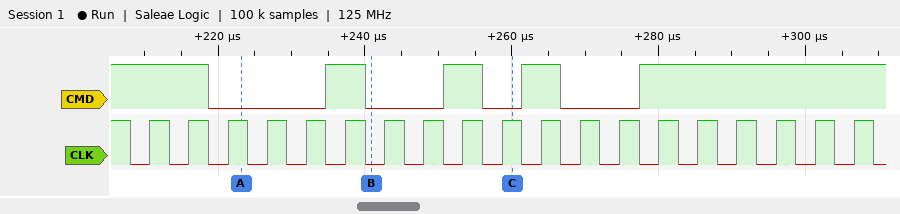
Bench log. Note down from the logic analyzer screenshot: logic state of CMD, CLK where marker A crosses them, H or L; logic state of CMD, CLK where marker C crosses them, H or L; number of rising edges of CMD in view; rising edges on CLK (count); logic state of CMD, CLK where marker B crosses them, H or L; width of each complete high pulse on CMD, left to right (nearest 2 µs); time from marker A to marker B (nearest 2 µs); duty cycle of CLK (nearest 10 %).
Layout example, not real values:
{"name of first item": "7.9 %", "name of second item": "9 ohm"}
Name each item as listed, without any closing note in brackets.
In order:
{"logic state of CMD, CLK where marker A crosses them, H or L": "CMD=L, CLK=H", "logic state of CMD, CLK where marker C crosses them, H or L": "CMD=L, CLK=H", "number of rising edges of CMD in view": "4", "rising edges on CLK": "19", "logic state of CMD, CLK where marker B crosses them, H or L": "CMD=L, CLK=L", "width of each complete high pulse on CMD, left to right": "6 µs, 6 µs, 6 µs", "time from marker A to marker B": "18 µs", "duty cycle of CLK": "50 %"}
